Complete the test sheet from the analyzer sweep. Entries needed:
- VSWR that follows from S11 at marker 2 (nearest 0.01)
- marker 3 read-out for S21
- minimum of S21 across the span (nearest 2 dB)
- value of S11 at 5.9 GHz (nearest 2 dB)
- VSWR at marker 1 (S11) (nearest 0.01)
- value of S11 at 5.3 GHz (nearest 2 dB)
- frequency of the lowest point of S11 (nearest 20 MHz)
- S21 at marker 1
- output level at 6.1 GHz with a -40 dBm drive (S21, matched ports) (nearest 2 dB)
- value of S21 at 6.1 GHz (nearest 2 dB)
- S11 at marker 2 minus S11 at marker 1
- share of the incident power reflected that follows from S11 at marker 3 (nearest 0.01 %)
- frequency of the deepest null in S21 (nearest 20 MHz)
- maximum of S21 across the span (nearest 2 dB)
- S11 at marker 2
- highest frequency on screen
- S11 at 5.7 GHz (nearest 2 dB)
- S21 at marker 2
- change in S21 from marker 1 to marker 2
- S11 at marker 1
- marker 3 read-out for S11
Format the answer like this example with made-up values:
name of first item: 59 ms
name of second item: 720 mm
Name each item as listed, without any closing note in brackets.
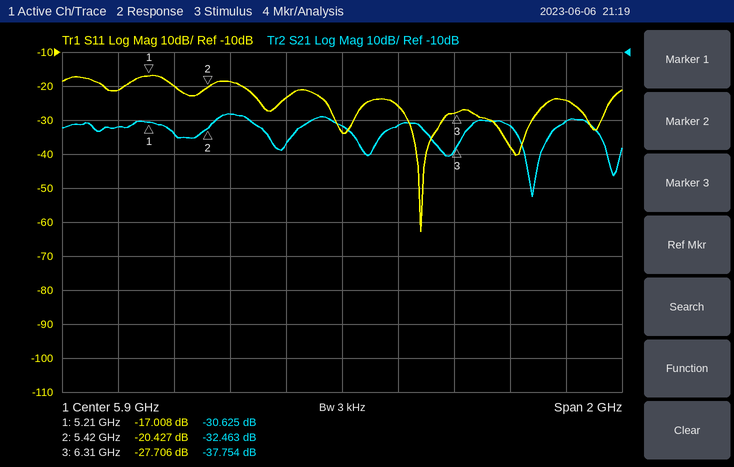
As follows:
VSWR that follows from S11 at marker 2: 1.21
marker 3 read-out for S21: -37.754 dB
minimum of S21 across the span: -52 dB
value of S11 at 5.9 GHz: -34 dB
VSWR at marker 1 (S11): 1.33
value of S11 at 5.3 GHz: -20 dB
frequency of the lowest point of S11: 6.18 GHz
S21 at marker 1: -30.625 dB
output level at 6.1 GHz with a -40 dBm drive (S21, matched ports): -72 dBm
value of S21 at 6.1 GHz: -32 dB
S11 at marker 2 minus S11 at marker 1: -3.419 dB
share of the incident power reflected that follows from S11 at marker 3: 0.17 %
frequency of the deepest null in S21: 6.58 GHz
maximum of S21 across the span: -28 dB
S11 at marker 2: -20.427 dB
highest frequency on screen: 6.9 GHz
S11 at 5.7 GHz: -24 dB
S21 at marker 2: -32.463 dB
change in S21 from marker 1 to marker 2: -1.838 dB
S11 at marker 1: -17.008 dB
marker 3 read-out for S11: -27.706 dB
